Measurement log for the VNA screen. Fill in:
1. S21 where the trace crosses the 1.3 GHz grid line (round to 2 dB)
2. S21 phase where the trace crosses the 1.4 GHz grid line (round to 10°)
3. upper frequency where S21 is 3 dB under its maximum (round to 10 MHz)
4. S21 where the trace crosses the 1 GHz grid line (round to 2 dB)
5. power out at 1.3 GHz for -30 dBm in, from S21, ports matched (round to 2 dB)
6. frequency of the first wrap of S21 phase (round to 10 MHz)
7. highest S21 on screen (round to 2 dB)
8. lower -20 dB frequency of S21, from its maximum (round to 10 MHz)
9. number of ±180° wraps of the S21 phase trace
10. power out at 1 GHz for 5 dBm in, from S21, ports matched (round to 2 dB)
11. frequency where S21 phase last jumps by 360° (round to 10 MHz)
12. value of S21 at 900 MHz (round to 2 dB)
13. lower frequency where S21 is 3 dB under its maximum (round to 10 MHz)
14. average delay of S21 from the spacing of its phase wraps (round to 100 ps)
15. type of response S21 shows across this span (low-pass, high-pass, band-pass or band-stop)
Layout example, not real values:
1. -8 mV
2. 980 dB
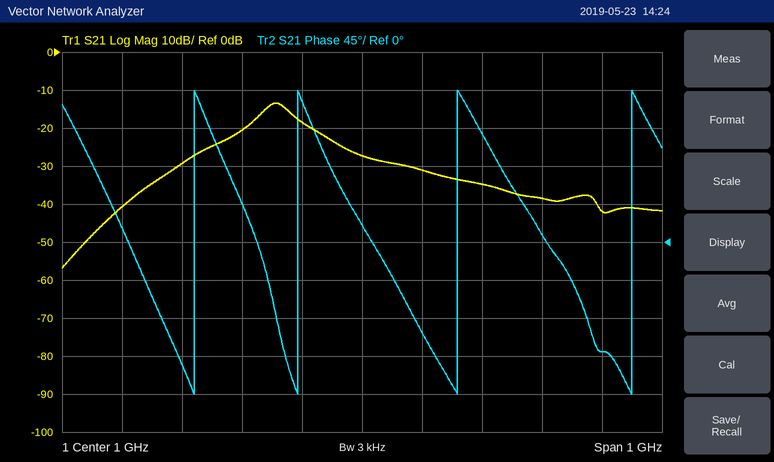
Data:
1. -38 dB
2. -130°
3. 880 MHz
4. -28 dB
5. -68 dBm
6. 720 MHz
7. -14 dB
8. 660 MHz
9. 4
10. -22 dBm
11. 1.45 GHz
12. -18 dB
13. 830 MHz
14. 4.1 ns
15. band-pass
